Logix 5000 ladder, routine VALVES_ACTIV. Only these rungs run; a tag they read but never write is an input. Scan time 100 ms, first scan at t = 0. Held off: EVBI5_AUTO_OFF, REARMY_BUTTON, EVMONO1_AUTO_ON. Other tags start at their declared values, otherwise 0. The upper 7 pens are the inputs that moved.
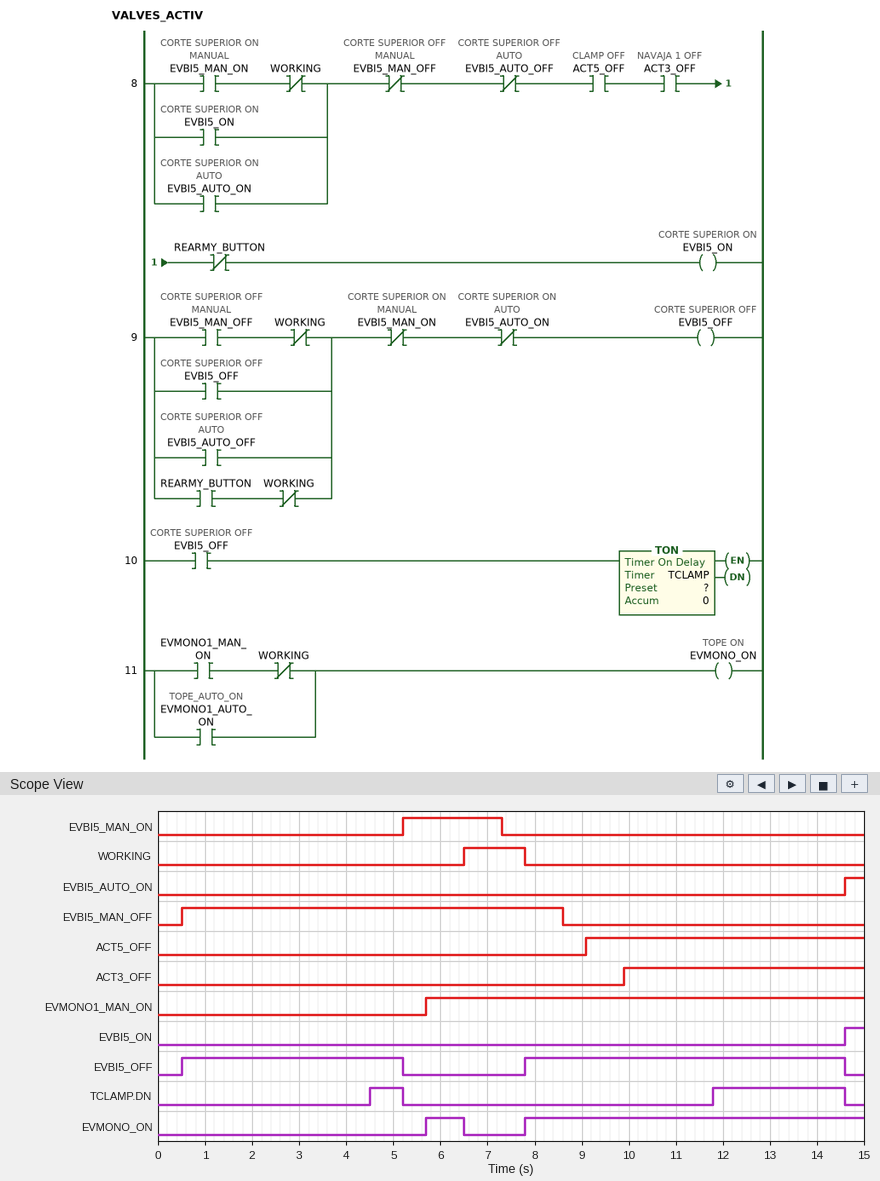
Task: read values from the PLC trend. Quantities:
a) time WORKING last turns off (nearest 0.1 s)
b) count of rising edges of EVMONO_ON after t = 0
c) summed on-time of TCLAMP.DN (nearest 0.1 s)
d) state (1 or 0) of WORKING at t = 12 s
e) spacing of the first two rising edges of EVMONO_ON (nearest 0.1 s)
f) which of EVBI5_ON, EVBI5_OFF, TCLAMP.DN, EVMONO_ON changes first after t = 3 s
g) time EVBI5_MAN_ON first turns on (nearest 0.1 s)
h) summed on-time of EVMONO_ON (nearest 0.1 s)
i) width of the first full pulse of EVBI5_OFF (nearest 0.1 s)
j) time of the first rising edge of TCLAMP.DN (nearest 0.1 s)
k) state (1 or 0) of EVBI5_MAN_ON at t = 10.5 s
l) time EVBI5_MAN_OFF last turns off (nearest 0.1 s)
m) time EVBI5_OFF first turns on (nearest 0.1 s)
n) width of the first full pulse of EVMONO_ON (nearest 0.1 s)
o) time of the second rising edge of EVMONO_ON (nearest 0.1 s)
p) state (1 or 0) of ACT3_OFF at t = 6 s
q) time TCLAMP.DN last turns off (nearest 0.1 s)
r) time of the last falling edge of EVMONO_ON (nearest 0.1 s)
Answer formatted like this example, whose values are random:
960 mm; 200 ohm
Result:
7.8 s; 2; 3.5 s; 0; 2.1 s; TCLAMP.DN; 5.2 s; 8.0 s; 4.7 s; 4.5 s; 0; 8.6 s; 0.5 s; 0.8 s; 7.8 s; 0; 14.6 s; 6.5 s
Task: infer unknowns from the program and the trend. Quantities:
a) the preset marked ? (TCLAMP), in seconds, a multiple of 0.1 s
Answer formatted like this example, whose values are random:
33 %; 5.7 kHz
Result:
4.0 s
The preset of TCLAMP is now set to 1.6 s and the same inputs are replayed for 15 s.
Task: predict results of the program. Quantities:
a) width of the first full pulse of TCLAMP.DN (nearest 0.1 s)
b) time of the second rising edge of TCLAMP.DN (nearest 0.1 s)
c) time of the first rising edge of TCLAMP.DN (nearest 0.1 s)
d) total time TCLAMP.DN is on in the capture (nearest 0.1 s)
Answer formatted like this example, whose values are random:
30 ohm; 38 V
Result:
3.1 s; 9.4 s; 2.1 s; 8.3 s
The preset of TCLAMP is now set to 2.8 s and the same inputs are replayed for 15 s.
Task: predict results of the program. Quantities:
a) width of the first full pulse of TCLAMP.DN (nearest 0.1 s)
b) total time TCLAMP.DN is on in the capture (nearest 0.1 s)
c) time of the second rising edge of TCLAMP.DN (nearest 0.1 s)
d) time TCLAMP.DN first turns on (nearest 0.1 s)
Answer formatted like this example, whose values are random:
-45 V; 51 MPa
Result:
1.9 s; 5.9 s; 10.6 s; 3.3 s
